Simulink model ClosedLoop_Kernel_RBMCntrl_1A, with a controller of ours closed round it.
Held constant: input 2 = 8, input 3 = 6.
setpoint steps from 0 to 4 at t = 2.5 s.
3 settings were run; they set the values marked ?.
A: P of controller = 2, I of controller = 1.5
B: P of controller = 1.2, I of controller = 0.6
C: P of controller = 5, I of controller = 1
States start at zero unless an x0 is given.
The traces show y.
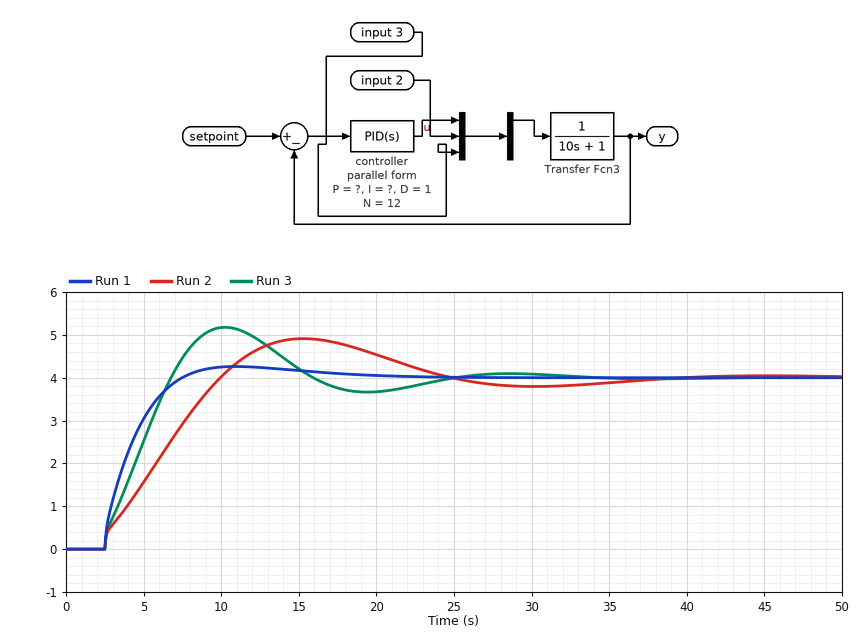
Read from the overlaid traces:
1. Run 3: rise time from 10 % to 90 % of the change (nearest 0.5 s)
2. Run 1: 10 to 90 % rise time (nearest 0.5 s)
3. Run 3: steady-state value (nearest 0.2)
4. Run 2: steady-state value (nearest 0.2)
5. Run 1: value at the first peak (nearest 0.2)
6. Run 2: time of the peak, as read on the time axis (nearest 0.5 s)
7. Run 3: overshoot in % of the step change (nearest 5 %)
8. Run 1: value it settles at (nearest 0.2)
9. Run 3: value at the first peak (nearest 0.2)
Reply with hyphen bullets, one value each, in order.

- 3.5 s
- 3.5 s
- 4.0
- 4.0
- 4.2
- 15.5 s
- 30 %
- 4.0
- 5.2
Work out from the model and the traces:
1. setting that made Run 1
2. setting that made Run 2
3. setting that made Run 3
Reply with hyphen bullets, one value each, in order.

- C
- B
- A
